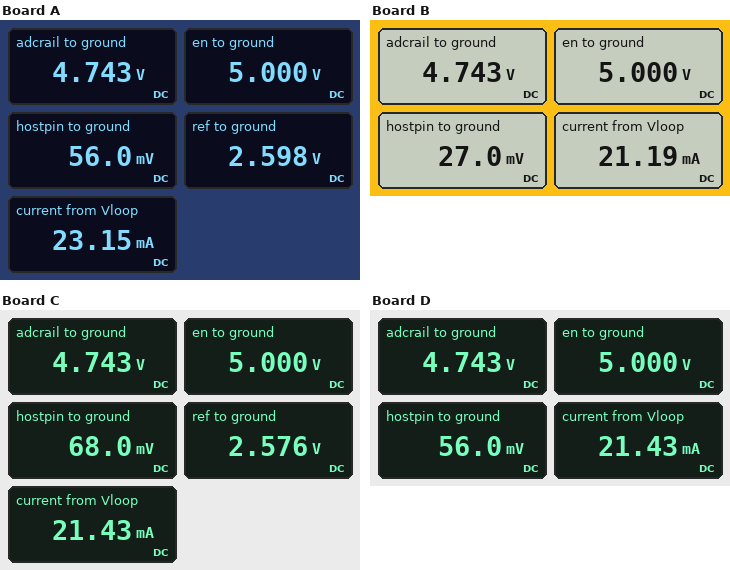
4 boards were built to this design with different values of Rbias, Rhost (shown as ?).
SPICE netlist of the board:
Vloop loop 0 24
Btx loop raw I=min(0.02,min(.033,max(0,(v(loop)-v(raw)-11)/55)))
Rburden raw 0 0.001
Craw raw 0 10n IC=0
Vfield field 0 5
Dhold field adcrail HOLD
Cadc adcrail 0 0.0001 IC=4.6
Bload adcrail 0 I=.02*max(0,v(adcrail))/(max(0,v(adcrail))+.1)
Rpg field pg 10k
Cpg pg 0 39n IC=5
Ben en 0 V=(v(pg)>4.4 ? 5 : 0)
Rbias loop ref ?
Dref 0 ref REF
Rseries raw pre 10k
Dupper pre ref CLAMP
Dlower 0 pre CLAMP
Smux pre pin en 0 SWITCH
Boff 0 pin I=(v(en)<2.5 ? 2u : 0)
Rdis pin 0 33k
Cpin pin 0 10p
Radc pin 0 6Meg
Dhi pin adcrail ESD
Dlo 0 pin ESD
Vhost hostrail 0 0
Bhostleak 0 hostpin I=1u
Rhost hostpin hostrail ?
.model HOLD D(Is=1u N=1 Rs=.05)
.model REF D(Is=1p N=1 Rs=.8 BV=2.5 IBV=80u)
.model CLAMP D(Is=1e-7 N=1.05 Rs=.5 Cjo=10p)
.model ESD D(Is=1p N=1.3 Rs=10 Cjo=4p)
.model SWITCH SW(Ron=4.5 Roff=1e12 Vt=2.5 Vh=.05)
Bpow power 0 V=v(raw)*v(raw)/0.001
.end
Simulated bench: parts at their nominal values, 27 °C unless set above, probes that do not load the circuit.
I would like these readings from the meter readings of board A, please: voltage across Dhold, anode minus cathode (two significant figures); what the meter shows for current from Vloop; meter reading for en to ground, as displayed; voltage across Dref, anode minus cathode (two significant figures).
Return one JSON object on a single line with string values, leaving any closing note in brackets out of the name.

{"voltage across Dhold, anode minus cathode": "260 mV", "what the meter shows for current from Vloop": "23.15 mA", "meter reading for en to ground, as displayed": "5.000 V", "voltage across Dref, anode minus cathode": "-2.6 V"}
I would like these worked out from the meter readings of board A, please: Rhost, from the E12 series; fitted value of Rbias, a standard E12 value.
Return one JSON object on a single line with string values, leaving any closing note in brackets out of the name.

{"Rhost, from the E12 series": "56 kΩ", "fitted value of Rbias, a standard E12 value": "6.8 kΩ"}
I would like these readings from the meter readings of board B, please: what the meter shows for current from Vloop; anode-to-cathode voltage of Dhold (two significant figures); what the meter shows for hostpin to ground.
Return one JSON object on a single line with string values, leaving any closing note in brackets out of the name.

{"what the meter shows for current from Vloop": "21.19 mA", "anode-to-cathode voltage of Dhold": "260 mV", "what the meter shows for hostpin to ground": "27.0 mV"}
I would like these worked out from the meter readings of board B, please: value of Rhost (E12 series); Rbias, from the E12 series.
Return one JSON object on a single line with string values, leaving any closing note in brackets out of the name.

{"value of Rhost": "27 kΩ", "Rbias, from the E12 series": "18 kΩ"}
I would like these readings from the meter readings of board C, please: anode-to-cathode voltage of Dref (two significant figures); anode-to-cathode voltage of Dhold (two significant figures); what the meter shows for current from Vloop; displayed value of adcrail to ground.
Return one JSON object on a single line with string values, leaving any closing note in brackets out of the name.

{"anode-to-cathode voltage of Dref": "-2.6 V", "anode-to-cathode voltage of Dhold": "260 mV", "what the meter shows for current from Vloop": "21.43 mA", "displayed value of adcrail to ground": "4.743 V"}
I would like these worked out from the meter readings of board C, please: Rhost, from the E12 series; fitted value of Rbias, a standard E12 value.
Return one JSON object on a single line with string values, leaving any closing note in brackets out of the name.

{"Rhost, from the E12 series": "68 kΩ", "fitted value of Rbias, a standard E12 value": "15 kΩ"}
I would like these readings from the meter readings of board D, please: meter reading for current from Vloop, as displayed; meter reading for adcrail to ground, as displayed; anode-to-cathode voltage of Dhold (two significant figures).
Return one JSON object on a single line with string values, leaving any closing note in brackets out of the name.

{"meter reading for current from Vloop, as displayed": "21.43 mA", "meter reading for adcrail to ground, as displayed": "4.743 V", "anode-to-cathode voltage of Dhold": "260 mV"}
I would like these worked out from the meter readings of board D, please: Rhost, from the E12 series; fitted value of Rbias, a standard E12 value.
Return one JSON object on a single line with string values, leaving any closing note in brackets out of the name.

{"Rhost, from the E12 series": "56 kΩ", "fitted value of Rbias, a standard E12 value": "15 kΩ"}
